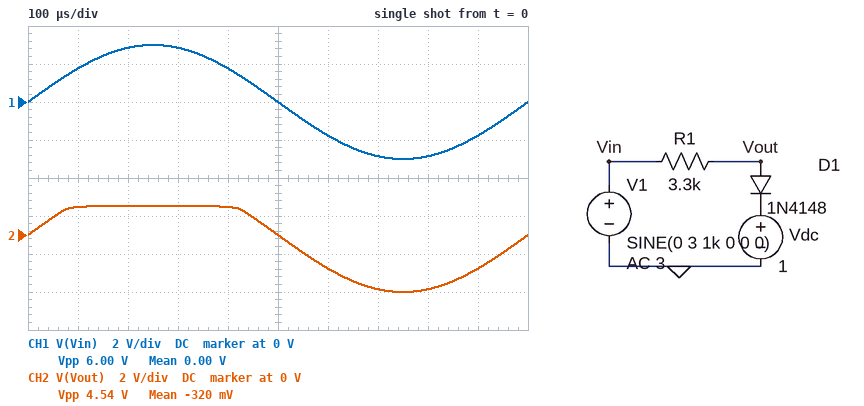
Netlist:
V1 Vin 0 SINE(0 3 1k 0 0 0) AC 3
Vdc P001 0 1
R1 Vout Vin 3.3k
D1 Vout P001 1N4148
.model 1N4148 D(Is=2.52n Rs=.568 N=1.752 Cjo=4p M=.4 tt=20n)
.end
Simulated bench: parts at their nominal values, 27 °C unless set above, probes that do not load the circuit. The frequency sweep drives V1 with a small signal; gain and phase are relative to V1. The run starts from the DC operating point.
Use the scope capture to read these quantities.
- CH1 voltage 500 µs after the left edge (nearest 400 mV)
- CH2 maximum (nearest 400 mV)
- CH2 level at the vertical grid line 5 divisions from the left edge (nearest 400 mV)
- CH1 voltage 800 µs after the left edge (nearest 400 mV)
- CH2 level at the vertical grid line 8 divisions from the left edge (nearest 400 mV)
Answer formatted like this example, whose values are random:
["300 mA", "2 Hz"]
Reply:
["0 V", "1.6 V", "0 V", "-2.8 V", "-2.8 V"]
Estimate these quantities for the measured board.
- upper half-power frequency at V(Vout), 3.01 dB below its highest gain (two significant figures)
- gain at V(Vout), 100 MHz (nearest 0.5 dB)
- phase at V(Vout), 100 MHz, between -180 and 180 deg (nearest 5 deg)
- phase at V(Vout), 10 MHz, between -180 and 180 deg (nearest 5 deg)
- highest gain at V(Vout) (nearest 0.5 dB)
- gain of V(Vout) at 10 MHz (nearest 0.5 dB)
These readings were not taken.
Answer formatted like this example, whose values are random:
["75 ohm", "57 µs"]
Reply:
["16 MHz", "-16.0 dB", "-80 deg", "-30 deg", "0 dB", "-1.5 dB"]
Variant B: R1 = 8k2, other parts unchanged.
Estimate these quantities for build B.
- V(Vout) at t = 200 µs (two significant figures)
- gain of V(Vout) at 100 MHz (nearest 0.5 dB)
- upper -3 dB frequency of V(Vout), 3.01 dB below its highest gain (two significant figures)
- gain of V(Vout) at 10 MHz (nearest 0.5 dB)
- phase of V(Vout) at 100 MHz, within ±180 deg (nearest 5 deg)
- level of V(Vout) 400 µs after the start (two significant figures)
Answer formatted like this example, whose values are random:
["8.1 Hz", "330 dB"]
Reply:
["1.5 V", "-24.0 dB", "6.4 MHz", "-5.5 dB", "-85 deg", "1.4 V"]
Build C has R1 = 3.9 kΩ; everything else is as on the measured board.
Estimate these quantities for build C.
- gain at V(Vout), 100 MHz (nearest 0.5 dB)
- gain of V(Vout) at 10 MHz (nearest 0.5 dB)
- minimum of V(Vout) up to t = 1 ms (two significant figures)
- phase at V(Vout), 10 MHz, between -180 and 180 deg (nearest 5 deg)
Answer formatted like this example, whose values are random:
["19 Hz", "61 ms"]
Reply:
["-17.5 dB", "-2.0 dB", "-3.0 V", "-35 deg"]
